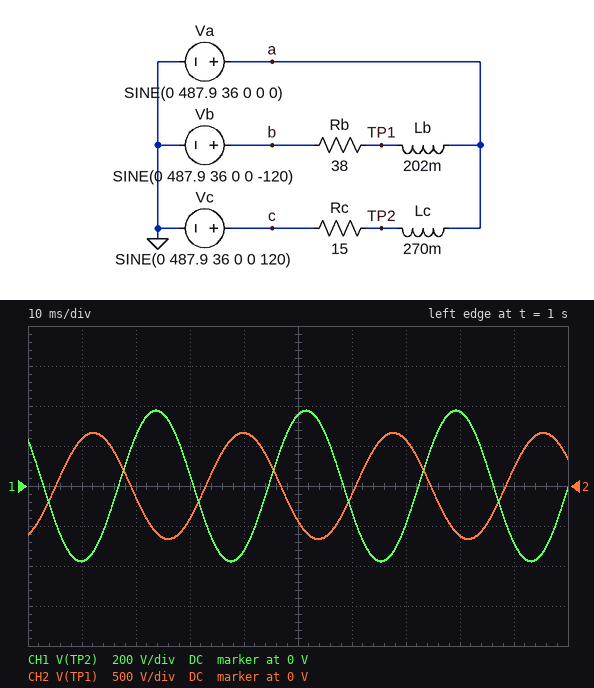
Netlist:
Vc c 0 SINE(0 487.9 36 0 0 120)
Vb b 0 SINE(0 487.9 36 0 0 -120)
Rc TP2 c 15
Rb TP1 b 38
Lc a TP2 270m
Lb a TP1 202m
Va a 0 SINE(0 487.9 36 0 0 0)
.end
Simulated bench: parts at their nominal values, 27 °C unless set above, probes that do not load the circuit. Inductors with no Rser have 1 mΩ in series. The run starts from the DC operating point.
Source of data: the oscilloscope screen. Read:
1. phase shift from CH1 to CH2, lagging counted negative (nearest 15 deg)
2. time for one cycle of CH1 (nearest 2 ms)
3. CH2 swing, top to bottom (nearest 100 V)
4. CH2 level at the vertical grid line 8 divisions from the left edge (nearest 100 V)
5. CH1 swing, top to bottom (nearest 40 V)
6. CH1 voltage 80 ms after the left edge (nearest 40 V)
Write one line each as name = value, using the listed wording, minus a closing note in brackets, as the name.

phase shift from CH1 to CH2, lagging counted negative = 150 deg
time for one cycle of CH1 = 28 ms
CH2 swing, top to bottom = 1.3 kV
CH2 level at the vertical grid line 8 divisions from the left edge = -600 V
CH1 swing, top to bottom = 760 V
CH1 voltage 80 ms after the left edge = 360 V
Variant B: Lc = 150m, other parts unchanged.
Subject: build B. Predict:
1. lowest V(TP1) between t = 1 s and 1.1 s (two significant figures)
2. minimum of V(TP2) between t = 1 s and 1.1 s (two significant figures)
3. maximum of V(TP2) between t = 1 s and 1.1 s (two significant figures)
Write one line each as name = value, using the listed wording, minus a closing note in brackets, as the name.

lowest V(TP1) between t = 1 s and 1.1 s = -660 V
minimum of V(TP2) between t = 1 s and 1.1 s = -290 V
maximum of V(TP2) between t = 1 s and 1.1 s = 290 V
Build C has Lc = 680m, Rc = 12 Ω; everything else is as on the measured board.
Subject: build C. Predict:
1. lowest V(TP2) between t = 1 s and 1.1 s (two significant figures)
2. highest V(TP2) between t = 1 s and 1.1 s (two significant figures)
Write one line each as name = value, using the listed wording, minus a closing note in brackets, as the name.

lowest V(TP2) between t = 1 s and 1.1 s = -450 V
highest V(TP2) between t = 1 s and 1.1 s = 450 V
